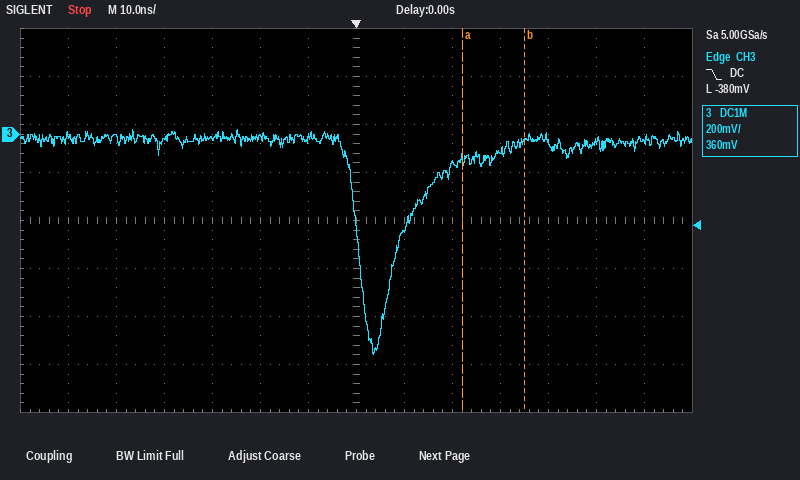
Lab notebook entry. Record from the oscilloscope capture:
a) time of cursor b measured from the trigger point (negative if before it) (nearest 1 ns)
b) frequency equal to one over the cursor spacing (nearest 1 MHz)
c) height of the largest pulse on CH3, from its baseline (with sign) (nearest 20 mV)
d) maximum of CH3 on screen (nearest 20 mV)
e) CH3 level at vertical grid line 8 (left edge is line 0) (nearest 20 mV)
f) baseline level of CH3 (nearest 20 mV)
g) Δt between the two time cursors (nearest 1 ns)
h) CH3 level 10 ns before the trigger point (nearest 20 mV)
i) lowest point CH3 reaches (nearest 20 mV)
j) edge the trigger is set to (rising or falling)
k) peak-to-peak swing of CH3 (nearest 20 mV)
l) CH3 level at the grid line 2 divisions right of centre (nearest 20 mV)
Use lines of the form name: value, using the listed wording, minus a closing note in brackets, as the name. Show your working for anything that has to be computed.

time of cursor b measured from the trigger point (negative if before it): +35 ns
frequency equal to one over the cursor spacing: 1 / 13 ns ≈ 77 MHz
height of the largest pulse on CH3, from its baseline (with sign): -920 mV − (-20 mV) = -900 mV
maximum of CH3 on screen: 20 mV
CH3 level at vertical grid line 8 (left edge is line 0): -400 mV
baseline level of CH3: -20 mV
Δt between the two time cursors: 13 ns
CH3 level 10 ns before the trigger point: -20 mV
lowest point CH3 reaches: -920 mV
edge the trigger is set to: falling
peak-to-peak swing of CH3: 20 mV − (-920 mV) = 940 mV
CH3 level at the grid line 2 divisions right of centre: -120 mV
